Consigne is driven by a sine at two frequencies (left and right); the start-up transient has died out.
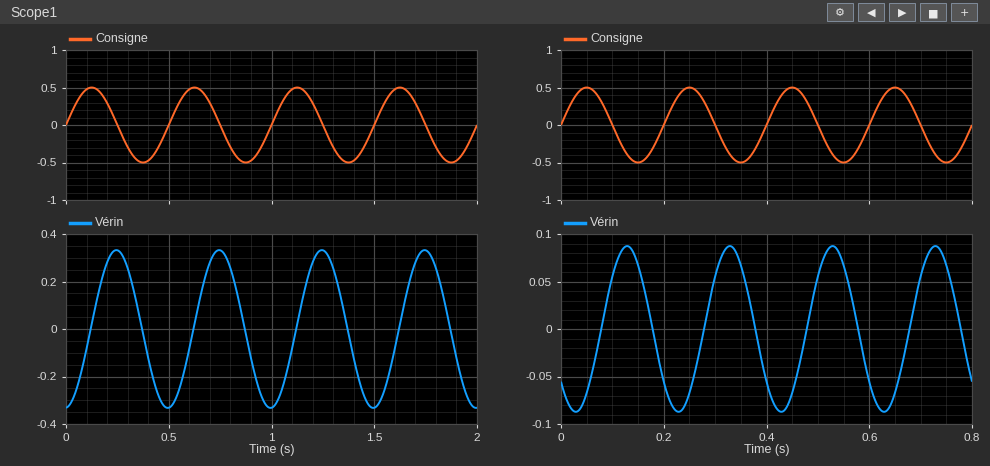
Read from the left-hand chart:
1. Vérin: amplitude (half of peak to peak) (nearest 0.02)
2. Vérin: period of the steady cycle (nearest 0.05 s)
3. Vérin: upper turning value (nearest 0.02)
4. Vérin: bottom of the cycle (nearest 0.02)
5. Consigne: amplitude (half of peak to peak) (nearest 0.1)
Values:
0.34
0.50 s
0.34
-0.34
0.5
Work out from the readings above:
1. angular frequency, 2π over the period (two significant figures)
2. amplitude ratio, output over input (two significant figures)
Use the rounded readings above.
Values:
13 rad/s
0.68
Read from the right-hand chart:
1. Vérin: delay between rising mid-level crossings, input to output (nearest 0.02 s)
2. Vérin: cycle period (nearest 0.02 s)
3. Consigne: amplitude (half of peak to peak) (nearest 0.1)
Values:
0.08 s
0.20 s
0.5
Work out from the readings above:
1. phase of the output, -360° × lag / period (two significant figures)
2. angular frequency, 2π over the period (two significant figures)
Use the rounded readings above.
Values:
-140°
31 rad/s
